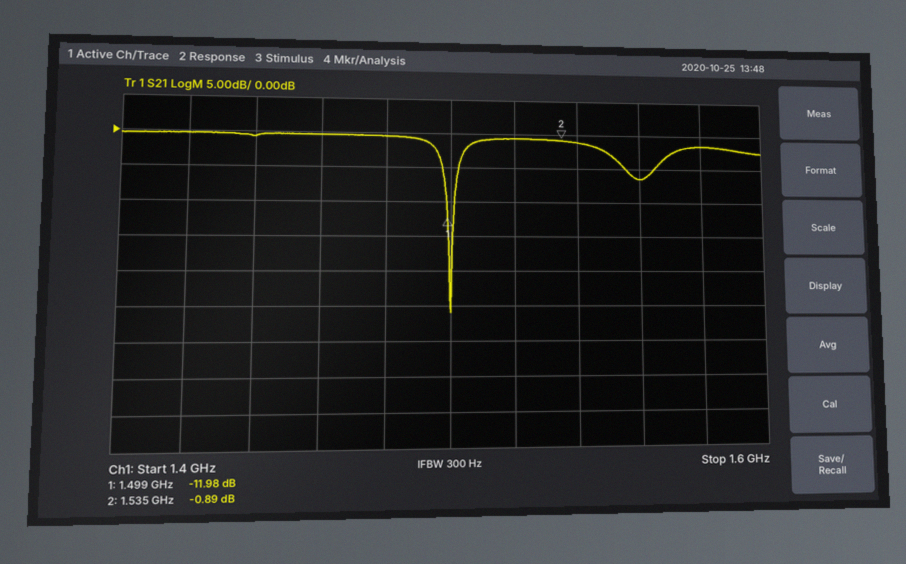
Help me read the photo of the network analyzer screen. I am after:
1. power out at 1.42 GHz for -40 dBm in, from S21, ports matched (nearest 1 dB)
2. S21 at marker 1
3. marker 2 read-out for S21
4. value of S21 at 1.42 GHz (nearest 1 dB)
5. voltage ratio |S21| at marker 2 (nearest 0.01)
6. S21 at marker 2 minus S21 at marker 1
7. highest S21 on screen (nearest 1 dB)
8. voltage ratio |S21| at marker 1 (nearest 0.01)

-40 dBm
-11.98 dB
-0.89 dB
0 dB
0.90
11.09 dB
0 dB
0.25
